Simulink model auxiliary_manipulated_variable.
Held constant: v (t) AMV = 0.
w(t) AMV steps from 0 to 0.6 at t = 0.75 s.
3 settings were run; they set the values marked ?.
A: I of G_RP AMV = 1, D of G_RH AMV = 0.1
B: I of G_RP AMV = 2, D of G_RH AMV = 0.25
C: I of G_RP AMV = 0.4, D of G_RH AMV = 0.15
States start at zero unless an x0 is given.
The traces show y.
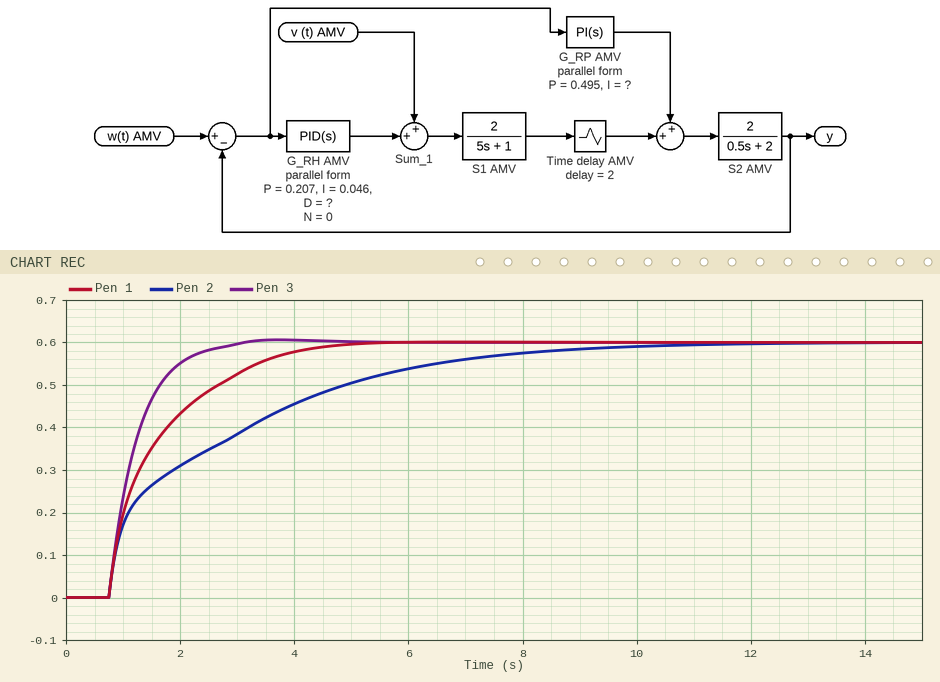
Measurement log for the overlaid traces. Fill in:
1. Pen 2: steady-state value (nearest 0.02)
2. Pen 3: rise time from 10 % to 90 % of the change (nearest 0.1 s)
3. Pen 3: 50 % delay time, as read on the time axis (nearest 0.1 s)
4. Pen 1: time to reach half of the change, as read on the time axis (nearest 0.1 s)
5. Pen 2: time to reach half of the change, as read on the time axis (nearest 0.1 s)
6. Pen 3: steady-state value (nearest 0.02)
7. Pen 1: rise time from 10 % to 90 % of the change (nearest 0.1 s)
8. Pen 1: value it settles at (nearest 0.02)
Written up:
0.60
1.1 s
1.1 s
1.3 s
1.9 s
0.60
2.4 s
0.60
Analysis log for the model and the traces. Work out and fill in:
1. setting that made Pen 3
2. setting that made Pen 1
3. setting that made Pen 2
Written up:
B
A
C
